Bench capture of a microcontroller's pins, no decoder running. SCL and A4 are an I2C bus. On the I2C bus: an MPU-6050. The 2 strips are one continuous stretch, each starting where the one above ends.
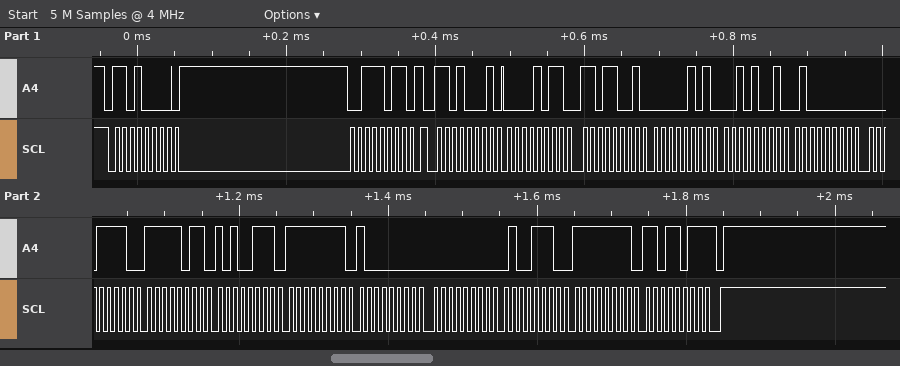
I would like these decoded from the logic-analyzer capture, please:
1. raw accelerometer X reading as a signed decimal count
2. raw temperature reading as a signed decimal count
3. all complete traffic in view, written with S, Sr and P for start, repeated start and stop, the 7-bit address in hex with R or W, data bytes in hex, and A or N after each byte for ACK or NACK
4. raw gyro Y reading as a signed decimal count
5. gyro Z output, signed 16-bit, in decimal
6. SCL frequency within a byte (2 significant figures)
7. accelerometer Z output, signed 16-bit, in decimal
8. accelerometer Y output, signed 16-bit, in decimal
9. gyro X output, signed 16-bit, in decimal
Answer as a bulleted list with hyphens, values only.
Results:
- 3033
- -1113
- S 68W A 3B A Sr 68R A 0B A D9 A 05 A 29 A 40 A 1E A FB A A7 A FF A 80 A 00 A 4E A FF A DB N P
- 78
- -37
- 100 kHz
- 16414
- 1321
- -128
